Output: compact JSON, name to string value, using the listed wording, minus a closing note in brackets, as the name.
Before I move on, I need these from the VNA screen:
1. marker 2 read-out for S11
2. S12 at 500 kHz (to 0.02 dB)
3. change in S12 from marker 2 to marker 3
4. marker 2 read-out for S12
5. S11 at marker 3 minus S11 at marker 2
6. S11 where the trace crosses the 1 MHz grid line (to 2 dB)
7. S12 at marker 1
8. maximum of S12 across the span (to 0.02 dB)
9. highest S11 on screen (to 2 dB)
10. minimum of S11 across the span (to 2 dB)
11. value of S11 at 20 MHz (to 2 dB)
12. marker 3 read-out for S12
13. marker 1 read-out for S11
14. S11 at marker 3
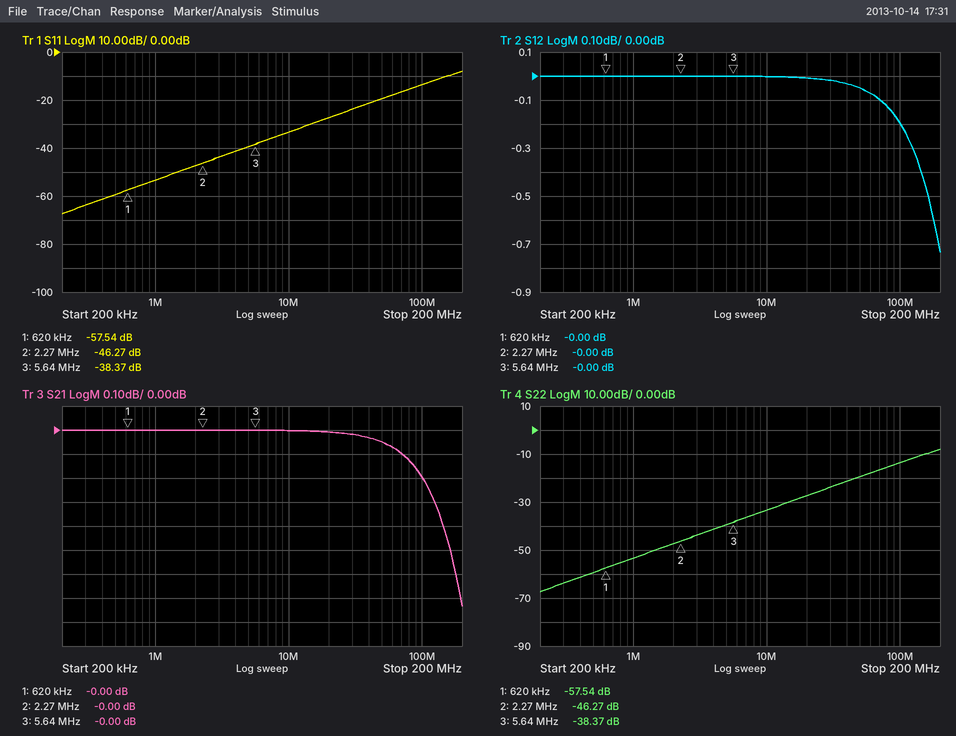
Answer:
{"marker 2 read-out for S11": "-46.27 dB", "S12 at 500 kHz": "0.00 dB", "change in S12 from marker 2 to marker 3": "0.00 dB", "marker 2 read-out for S12": "-0.00 dB", "S11 at marker 3 minus S11 at marker 2": "7.90 dB", "S11 where the trace crosses the 1 MHz grid line": "-54 dB", "S12 at marker 1": "-0.00 dB", "maximum of S12 across the span": "0.00 dB", "highest S11 on screen": "-8 dB", "minimum of S11 across the span": "-68 dB", "value of S11 at 20 MHz": "-28 dB", "marker 3 read-out for S12": "-0.00 dB", "marker 1 read-out for S11": "-57.54 dB", "S11 at marker 3": "-38.37 dB"}
